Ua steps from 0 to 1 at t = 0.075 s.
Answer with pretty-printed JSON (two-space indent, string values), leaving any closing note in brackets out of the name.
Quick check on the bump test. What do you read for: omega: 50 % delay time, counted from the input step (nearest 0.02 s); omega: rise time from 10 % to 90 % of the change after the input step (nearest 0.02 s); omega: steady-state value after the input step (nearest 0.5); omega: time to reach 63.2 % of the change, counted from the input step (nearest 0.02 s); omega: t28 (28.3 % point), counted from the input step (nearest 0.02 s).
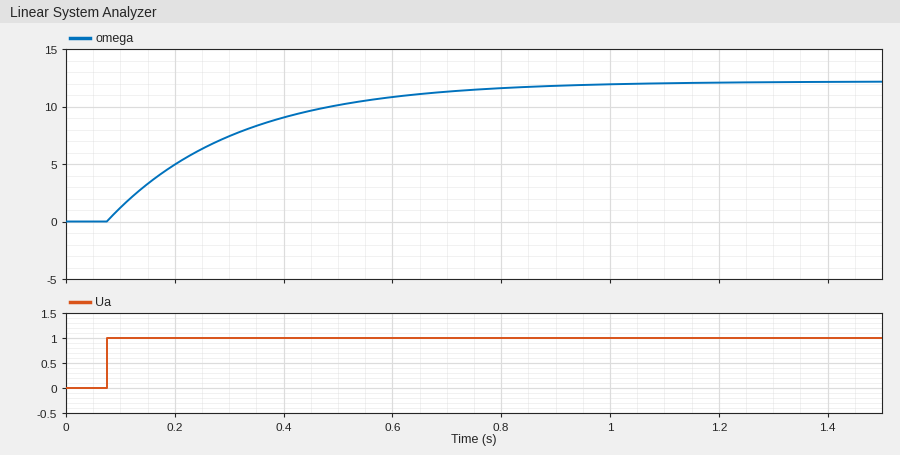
{
  "omega: 50 % delay time, counted from the input step": "0.16 s",
  "omega: rise time from 10 % to 90 % of the change after the input step": "0.52 s",
  "omega: steady-state value after the input step": "12.0",
  "omega: time to reach 63.2 % of the change, counted from the input step": "0.24 s",
  "omega: t28 (28.3 % point), counted from the input step": "0.08 s"
}
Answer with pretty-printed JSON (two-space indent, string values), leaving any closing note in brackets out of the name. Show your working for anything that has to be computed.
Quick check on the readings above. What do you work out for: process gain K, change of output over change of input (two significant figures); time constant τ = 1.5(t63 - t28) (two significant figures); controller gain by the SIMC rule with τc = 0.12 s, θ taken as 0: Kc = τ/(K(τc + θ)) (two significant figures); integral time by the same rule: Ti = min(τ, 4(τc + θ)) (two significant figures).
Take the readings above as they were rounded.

{
  "process gain K, change of output over change of input": "(12 - 0) / 1 = 12",
  "time constant τ = 1.5(t63 - t28)": "1.5 × (0.24 - 0.08) = 0.24 s",
  "controller gain by the SIMC rule with τc = 0.12 s, θ taken as 0: Kc = τ/(K(τc + θ))": "0.24 / (12 × (0.12 + 0)) = 0.17",
  "integral time by the same rule: Ti = min(τ, 4(τc + θ))": "min(0.24, 4 × (0.12 + 0)) = 0.24 s"
}
